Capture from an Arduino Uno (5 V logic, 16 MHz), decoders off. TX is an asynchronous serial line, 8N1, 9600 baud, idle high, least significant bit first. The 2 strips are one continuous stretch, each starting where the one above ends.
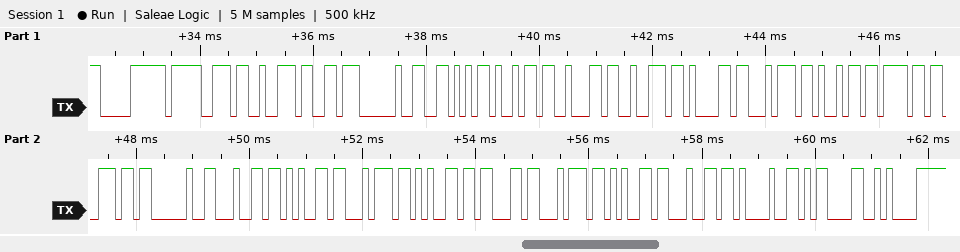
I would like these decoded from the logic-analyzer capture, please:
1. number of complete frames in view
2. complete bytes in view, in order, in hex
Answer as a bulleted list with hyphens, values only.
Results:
- 26
- F0 9F 93 B3 20 56 69 62 72 61 74 69 6F 6E 20 64 65 74 65 63 74 65 64 21 0D 0A
